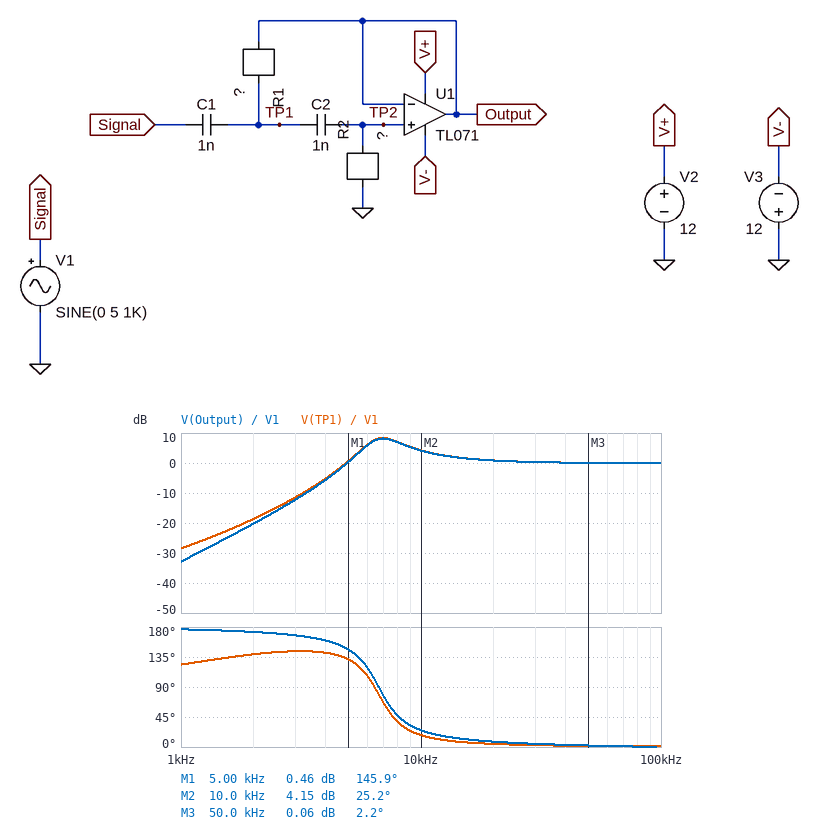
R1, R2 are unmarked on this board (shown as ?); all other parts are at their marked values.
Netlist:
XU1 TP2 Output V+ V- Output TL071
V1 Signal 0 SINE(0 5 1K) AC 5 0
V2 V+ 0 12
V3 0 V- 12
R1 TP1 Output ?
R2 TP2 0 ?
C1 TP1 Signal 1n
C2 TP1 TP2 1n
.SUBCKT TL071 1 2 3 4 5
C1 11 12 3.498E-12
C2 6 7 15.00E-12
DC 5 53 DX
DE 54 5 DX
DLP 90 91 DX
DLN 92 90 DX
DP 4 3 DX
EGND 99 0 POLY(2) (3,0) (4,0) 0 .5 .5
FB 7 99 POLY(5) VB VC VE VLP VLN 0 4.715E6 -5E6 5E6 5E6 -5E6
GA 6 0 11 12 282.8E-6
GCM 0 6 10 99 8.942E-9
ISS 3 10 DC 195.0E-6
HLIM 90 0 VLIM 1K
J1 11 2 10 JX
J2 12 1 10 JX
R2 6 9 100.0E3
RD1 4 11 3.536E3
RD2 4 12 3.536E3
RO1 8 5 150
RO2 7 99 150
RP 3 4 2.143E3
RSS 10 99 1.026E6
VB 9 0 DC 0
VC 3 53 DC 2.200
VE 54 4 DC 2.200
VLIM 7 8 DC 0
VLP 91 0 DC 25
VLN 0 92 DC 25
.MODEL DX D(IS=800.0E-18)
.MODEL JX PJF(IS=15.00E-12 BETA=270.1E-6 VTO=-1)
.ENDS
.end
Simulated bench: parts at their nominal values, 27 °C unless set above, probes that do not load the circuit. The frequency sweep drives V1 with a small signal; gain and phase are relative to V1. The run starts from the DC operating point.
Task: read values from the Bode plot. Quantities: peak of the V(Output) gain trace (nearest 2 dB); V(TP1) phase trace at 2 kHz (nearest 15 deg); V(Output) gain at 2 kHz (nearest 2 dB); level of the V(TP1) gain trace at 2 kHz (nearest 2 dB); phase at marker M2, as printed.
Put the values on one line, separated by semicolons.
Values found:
8 dB; 135 deg; -20 dB; -18 dB; 25.2 deg
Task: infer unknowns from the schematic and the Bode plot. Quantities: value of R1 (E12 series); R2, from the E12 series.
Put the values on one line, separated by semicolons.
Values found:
4.7 kΩ; 120 kΩ
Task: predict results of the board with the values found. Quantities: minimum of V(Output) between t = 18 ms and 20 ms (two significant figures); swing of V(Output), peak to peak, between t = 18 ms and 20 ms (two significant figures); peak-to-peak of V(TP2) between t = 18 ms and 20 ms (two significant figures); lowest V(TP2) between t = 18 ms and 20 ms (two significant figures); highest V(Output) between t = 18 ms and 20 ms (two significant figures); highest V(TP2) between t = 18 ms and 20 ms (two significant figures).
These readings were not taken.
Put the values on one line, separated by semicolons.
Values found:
-110 mV; 230 mV; 230 mV; -110 mV; 110 mV; 110 mV
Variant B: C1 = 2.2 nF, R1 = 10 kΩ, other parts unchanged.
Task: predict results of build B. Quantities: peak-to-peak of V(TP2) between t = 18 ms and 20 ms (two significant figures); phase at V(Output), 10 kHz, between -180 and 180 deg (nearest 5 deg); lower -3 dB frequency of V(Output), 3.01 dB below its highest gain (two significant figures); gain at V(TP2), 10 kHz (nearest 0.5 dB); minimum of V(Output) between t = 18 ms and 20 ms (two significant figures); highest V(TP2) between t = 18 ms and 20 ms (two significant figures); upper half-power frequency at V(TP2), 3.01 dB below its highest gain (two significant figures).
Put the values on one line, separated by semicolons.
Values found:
1.1 V; 10 deg; 2.6 kHz; 0.5 dB; -570 mV; 570 mV; 6.7 kHz
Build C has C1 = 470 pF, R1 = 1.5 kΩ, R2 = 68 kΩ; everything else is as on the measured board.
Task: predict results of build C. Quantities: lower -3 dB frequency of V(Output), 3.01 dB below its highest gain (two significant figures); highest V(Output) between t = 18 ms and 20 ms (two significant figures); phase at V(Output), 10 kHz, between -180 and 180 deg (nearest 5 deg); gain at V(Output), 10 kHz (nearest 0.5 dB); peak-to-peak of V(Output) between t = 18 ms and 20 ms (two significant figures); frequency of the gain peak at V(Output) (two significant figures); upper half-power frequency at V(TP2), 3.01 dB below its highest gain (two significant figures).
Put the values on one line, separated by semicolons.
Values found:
20 kHz; 9.5 mV; 170 deg; -12.5 dB; 19 mV; 23 kHz; 28 kHz
